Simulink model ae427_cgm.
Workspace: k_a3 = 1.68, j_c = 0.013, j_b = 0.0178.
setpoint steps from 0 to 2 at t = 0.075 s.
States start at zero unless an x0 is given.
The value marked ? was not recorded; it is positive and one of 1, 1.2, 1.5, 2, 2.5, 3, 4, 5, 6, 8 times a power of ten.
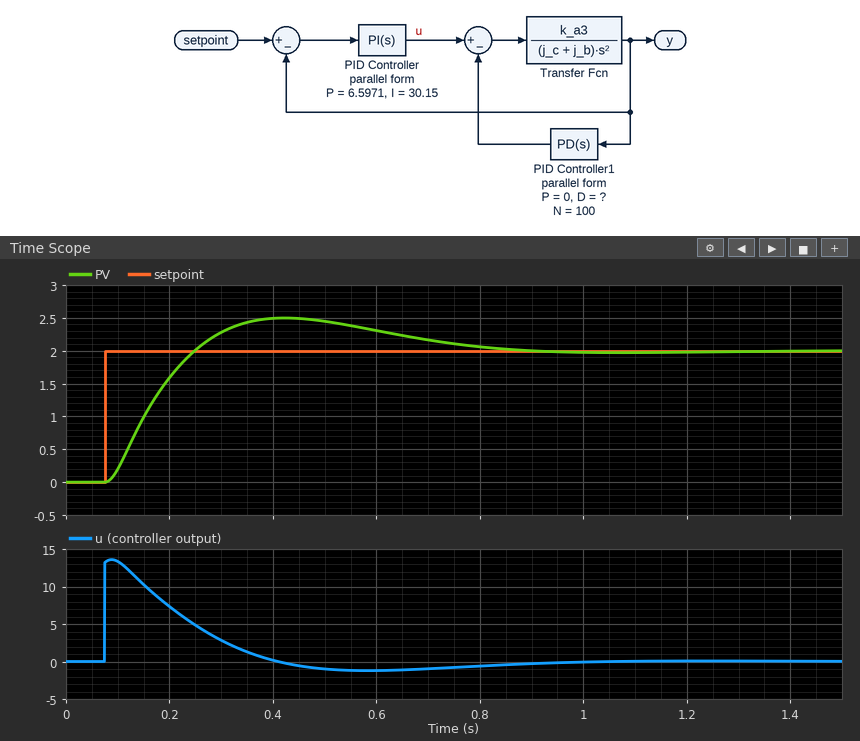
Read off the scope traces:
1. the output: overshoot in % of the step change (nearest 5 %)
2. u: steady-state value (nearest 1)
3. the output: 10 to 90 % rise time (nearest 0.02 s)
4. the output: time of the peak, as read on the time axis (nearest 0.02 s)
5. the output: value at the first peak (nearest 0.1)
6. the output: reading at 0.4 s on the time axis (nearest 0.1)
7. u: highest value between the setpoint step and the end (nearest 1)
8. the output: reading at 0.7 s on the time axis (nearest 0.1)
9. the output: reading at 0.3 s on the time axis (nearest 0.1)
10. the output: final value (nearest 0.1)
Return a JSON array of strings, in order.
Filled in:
["25 %", "0", "0.12 s", "0.42 s", "2.5", "2.5", "14", "2.2", "2.3", "2.0"]
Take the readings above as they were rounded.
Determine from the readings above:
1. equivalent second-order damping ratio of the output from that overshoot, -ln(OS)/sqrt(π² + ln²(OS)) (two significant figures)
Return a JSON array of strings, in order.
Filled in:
["0.40"]
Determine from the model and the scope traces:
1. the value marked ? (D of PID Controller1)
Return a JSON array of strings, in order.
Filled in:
["0.8"]
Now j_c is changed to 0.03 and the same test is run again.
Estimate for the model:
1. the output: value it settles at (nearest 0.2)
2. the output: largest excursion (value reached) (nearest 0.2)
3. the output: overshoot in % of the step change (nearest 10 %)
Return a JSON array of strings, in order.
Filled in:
["2.0", "2.6", "30 %"]
